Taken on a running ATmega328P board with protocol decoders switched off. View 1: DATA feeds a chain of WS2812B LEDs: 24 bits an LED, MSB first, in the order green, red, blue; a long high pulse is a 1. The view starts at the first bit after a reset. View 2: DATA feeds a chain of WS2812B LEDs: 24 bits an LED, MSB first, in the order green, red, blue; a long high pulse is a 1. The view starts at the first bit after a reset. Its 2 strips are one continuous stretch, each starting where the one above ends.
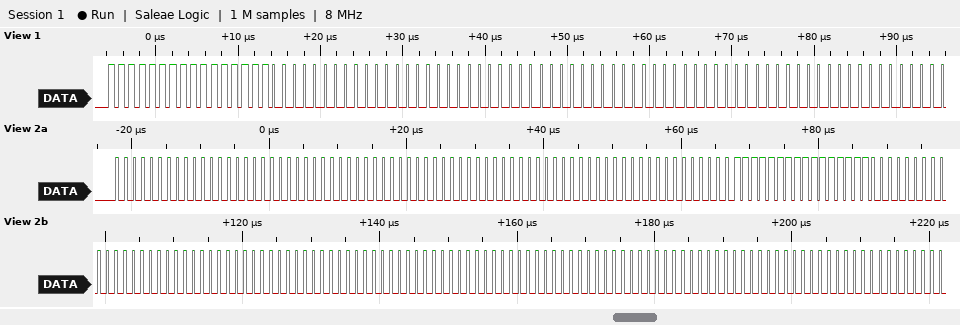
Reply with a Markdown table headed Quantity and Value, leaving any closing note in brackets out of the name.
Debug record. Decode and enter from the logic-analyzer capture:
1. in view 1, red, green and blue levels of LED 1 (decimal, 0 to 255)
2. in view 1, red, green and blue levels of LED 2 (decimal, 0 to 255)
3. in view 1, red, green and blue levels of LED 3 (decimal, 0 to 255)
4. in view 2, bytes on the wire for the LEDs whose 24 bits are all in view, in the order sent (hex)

| Quantity | Value |
|---|---|
| in view 1, red, green and blue levels of LED 1 | 255, 255, 0 |
| in view 1, red, green and blue levels of LED 2 | 0, 0, 0 |
| in view 1, red, green and blue levels of LED 3 | 0, 0, 0 |
| in view 2, bytes on the wire for the LEDs whose 24 bits are all in view, in the order sent | 00 00 00 00 00 00 00 00 00 FF FF 00 00 00 00 00 00 00 00 00 00 00 00 00 |
